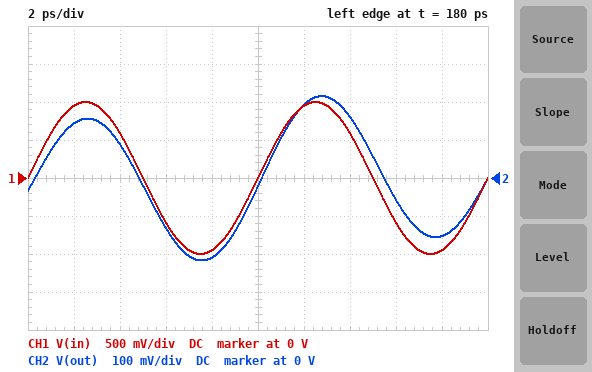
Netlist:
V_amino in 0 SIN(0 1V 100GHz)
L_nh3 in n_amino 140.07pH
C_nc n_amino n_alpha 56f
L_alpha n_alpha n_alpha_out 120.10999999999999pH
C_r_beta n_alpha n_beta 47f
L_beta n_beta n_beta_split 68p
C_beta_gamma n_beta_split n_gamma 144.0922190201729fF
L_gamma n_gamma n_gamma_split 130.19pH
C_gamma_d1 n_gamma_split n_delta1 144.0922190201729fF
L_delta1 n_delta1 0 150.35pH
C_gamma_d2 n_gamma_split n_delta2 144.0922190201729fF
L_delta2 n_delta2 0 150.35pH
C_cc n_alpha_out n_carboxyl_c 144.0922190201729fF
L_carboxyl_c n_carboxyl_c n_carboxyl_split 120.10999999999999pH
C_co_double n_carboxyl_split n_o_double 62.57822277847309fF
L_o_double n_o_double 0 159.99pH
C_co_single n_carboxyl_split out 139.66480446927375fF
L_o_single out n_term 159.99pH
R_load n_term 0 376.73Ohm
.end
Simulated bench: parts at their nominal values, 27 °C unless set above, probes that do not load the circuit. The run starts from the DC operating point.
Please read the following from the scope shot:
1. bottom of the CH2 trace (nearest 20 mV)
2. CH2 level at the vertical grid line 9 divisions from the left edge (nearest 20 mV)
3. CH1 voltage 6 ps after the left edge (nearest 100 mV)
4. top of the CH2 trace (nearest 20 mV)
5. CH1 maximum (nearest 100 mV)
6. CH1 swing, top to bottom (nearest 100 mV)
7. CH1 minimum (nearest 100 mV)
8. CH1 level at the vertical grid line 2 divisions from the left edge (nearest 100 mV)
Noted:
-220 mV
-160 mV
-600 mV
220 mV
1.0 V
2.0 V
-1.0 V
600 mV
